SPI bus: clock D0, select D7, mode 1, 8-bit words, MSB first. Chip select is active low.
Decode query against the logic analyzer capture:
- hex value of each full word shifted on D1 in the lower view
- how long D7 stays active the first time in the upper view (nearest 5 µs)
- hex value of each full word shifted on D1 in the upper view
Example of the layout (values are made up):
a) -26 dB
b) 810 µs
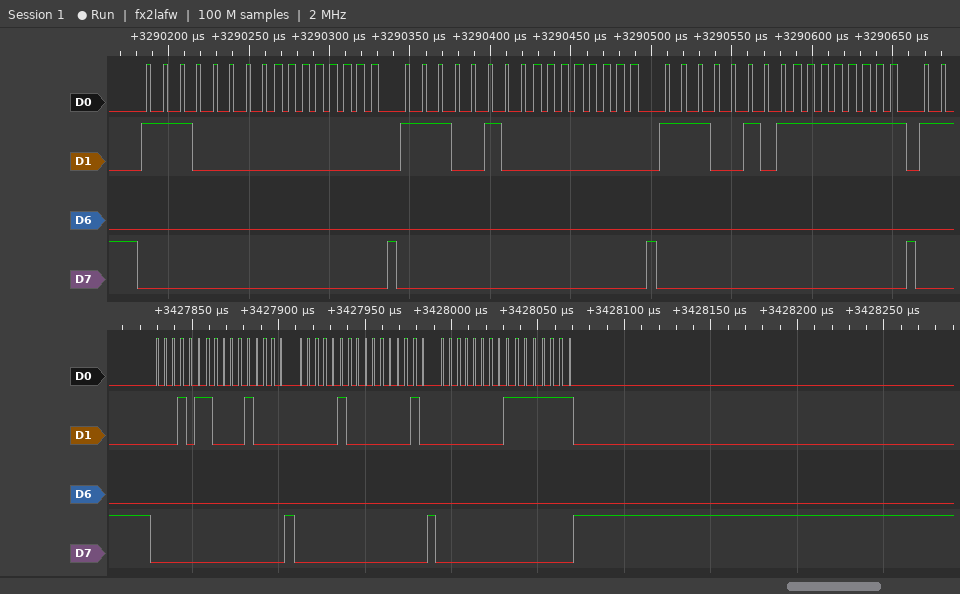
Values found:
a) 16, 10, 04, 02, 00, FF
b) 155 µs
c) E0, 00, E4, 00, E5, FF
